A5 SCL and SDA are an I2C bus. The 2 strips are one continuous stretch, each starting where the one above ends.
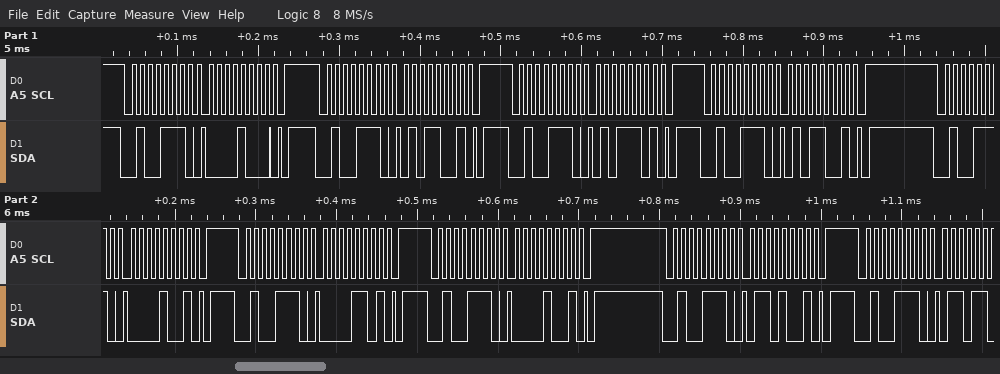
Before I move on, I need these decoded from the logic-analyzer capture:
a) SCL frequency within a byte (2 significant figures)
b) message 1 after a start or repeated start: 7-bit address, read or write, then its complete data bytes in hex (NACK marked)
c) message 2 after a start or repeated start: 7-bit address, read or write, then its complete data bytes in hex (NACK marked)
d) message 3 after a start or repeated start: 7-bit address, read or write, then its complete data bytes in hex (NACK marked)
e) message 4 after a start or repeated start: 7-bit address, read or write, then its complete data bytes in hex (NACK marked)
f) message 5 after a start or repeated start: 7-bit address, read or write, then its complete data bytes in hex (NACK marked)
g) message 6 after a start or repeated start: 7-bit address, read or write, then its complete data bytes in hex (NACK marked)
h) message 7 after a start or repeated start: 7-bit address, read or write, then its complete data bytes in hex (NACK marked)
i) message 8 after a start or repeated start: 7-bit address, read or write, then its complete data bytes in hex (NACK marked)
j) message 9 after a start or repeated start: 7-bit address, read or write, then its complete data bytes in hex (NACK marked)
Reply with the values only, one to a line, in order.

100 kHz
0x27 write: 08
0x27 write: 59
0x27 write: 5D
0x27 write: 59
0x27 write: 09
0x27 write: 0D
0x27 write: 09
0x27 write: 69
0x27 write
